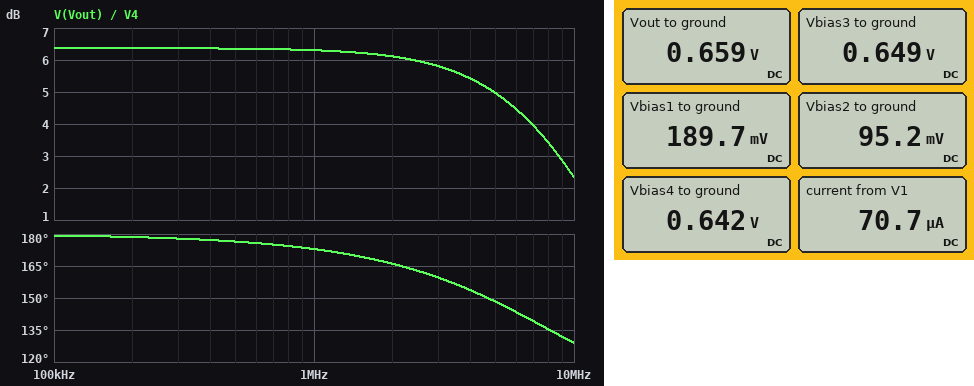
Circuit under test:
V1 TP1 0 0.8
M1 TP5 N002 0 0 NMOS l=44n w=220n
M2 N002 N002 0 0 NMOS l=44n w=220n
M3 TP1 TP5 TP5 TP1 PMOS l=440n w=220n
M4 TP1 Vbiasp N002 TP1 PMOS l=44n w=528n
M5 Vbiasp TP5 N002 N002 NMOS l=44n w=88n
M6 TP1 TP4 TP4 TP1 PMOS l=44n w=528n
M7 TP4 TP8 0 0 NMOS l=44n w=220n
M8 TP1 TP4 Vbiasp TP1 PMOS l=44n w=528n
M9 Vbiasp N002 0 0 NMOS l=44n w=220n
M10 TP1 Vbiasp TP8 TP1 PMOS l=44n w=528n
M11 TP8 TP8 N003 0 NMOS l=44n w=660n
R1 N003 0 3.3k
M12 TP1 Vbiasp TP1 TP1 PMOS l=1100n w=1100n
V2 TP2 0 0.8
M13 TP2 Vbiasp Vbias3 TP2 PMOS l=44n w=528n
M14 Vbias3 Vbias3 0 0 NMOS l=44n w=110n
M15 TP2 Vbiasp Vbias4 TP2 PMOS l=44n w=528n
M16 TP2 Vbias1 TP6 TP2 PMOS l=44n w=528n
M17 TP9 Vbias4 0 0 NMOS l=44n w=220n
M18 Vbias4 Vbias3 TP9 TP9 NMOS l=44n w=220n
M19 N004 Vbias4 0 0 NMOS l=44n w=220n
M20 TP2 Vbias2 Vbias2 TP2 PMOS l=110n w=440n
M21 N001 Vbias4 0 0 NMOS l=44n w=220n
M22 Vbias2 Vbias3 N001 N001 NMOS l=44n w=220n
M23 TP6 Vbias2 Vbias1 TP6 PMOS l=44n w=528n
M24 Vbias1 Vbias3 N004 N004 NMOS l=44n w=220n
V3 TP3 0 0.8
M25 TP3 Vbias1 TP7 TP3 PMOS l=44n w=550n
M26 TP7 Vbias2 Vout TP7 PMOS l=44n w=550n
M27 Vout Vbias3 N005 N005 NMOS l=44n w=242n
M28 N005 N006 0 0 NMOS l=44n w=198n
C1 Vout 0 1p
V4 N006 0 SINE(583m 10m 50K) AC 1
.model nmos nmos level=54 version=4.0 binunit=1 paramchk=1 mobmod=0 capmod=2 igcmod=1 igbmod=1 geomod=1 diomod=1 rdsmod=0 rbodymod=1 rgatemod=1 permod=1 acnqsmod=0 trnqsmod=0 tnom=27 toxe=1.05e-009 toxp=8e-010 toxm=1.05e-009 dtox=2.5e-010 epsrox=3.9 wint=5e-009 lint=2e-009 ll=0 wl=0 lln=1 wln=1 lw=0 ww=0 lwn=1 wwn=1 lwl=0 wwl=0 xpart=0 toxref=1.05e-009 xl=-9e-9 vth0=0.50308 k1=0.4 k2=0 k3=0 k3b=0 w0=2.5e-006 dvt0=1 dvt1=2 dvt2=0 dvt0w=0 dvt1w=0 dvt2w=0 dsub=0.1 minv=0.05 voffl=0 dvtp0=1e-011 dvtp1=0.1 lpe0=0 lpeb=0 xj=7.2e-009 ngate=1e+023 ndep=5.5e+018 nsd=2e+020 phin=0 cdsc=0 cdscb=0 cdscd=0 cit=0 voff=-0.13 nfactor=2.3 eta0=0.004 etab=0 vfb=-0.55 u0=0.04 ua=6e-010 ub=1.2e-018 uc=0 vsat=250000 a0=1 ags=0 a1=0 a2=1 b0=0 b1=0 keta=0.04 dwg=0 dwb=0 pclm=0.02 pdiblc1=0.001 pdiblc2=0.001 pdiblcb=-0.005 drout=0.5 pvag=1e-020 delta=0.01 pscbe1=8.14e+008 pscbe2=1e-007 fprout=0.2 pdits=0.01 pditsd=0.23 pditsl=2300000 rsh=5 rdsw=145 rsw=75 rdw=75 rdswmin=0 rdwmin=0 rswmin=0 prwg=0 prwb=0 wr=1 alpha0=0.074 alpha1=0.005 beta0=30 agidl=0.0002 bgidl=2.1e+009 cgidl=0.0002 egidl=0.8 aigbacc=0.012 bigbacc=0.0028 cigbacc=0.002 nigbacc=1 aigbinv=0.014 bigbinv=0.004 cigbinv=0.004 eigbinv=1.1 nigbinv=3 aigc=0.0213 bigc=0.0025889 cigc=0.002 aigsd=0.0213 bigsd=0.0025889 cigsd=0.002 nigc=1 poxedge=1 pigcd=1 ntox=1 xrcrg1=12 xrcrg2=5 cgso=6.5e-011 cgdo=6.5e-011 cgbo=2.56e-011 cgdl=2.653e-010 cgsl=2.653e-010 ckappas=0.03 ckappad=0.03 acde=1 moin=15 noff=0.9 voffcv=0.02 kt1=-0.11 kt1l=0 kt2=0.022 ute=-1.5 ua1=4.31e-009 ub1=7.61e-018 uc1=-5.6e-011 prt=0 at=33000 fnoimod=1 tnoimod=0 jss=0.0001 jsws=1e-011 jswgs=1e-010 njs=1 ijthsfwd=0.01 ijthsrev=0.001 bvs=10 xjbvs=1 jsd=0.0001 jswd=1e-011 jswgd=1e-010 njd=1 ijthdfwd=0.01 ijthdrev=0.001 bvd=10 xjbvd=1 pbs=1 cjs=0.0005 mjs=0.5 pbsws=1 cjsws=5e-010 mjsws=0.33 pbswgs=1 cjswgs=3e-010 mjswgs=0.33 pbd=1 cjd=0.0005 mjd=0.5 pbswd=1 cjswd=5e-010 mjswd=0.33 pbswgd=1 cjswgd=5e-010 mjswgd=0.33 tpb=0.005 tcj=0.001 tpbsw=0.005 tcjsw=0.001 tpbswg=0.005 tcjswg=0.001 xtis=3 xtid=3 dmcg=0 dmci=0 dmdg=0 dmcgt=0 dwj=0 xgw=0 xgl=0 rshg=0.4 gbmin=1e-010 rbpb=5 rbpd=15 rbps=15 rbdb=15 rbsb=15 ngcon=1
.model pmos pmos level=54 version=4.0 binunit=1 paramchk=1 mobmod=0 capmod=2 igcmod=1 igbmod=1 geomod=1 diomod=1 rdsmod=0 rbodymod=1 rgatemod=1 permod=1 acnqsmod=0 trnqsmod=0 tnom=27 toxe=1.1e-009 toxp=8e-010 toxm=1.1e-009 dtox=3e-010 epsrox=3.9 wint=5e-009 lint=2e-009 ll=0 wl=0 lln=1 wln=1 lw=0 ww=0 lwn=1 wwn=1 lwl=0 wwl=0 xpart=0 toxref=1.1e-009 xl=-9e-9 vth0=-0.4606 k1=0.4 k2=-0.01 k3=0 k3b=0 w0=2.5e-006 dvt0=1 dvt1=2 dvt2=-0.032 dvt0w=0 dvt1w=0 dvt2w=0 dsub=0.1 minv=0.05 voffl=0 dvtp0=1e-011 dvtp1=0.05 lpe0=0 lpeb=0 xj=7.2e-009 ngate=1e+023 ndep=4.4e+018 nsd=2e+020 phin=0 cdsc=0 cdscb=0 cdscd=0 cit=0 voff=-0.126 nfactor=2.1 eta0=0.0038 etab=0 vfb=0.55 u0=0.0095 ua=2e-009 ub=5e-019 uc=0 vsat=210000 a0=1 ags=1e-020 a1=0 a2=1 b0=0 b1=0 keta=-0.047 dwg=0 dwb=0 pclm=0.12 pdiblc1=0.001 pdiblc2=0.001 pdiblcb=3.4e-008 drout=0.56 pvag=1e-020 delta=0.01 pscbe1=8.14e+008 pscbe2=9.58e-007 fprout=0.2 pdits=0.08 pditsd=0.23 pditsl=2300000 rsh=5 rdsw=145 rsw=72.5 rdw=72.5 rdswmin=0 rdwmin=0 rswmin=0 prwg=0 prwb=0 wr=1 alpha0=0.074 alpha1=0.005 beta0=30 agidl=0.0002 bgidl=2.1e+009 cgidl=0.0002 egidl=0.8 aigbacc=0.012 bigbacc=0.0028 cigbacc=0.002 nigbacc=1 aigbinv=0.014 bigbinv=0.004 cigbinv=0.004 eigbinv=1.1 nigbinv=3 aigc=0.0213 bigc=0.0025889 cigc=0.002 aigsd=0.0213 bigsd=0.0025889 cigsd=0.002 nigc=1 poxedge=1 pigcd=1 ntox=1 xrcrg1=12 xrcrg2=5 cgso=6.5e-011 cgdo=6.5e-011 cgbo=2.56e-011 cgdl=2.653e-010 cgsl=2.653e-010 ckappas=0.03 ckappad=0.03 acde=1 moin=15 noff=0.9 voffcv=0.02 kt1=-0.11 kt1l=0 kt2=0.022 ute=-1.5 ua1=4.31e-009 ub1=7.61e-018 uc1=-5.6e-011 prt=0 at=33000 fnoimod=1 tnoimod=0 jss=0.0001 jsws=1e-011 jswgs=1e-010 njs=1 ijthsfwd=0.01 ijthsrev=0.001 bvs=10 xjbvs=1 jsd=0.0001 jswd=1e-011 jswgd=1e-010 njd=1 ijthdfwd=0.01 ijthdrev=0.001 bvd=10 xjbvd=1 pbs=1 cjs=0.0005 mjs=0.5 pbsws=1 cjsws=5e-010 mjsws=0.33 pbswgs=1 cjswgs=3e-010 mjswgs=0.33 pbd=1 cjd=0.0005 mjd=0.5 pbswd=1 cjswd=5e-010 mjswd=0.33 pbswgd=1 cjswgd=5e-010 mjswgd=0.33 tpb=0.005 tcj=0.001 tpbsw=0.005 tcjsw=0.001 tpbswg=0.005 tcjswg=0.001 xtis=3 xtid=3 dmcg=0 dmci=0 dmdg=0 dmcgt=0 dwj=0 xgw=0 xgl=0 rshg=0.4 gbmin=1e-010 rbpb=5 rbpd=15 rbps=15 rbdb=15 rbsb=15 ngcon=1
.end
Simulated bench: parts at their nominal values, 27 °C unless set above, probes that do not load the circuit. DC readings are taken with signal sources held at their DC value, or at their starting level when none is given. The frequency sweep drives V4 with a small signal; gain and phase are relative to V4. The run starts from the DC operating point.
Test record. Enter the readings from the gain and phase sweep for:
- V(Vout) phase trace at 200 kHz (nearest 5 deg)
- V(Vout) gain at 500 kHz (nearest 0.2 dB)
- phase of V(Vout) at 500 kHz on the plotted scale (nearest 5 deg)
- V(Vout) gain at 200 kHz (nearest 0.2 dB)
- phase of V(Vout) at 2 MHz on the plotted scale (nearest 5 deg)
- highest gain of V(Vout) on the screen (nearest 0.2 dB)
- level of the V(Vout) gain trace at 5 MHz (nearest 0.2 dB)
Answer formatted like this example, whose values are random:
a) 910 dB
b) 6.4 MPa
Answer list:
a) 180 deg
b) 6.4 dB
c) 175 deg
d) 6.4 dB
e) 165 deg
f) 6.4 dB
g) 5.0 dB
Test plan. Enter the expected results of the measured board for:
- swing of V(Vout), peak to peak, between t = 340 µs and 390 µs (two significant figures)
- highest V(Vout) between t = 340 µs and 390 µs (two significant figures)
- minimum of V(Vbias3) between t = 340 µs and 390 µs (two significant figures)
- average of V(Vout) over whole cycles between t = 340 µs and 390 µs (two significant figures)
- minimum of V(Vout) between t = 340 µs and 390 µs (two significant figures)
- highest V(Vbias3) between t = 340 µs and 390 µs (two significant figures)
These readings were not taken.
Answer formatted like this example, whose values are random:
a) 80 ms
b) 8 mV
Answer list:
a) 42 mV
b) 680 mV
c) 650 mV
d) 660 mV
e) 640 mV
f) 650 mV
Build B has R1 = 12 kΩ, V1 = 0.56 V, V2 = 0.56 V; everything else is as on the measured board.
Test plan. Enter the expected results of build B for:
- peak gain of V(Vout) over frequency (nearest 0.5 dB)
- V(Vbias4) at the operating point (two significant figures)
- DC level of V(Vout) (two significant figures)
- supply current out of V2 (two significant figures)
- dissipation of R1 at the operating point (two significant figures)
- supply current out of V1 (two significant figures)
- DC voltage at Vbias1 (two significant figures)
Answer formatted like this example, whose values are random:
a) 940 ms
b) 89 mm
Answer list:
a) -23.0 dB
b) 500 mV
c) 770 mV
d) 8.7 µA
e) 120 nW
f) 11 µA
g) 81 mV
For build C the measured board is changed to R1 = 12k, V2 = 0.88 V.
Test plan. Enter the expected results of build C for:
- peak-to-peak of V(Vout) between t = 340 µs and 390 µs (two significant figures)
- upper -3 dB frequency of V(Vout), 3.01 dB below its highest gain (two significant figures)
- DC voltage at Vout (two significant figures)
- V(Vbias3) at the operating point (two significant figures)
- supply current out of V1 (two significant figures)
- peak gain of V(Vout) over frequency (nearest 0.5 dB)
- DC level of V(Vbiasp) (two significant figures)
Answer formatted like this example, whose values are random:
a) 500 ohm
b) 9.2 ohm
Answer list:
a) 4.5 mV
b) 14 MHz
c) 38 mV
d) 620 mV
e) 17 µA
f) -13.0 dB
g) 310 mV
